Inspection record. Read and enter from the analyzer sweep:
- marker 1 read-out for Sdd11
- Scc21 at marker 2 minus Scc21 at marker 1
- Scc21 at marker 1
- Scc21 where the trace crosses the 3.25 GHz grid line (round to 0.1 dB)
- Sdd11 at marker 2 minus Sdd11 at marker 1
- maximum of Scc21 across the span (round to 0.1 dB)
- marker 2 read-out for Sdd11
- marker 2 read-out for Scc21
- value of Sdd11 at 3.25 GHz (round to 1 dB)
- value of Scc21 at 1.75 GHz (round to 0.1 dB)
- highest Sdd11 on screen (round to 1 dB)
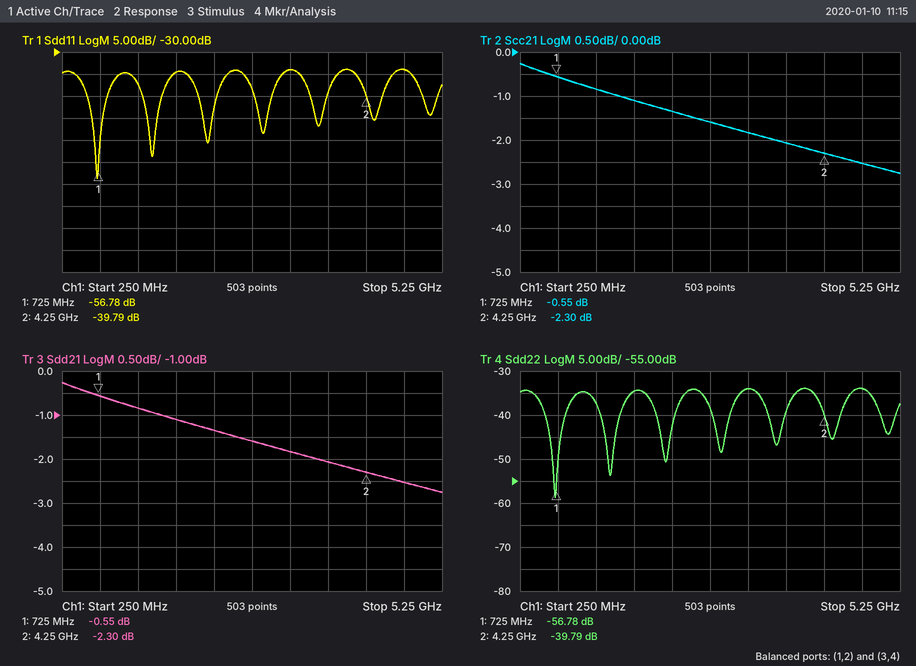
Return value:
-56.78 dB
-1.75 dB
-0.55 dB
-1.8 dB
16.99 dB
-0.3 dB
-39.79 dB
-2.30 dB
-34 dB
-1.1 dB
-34 dB
